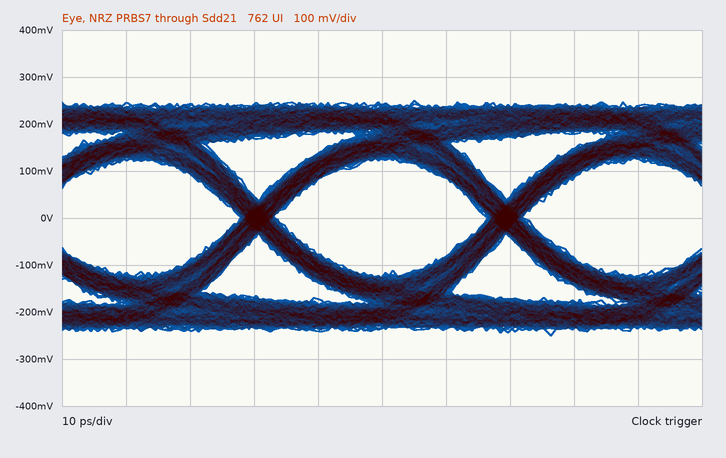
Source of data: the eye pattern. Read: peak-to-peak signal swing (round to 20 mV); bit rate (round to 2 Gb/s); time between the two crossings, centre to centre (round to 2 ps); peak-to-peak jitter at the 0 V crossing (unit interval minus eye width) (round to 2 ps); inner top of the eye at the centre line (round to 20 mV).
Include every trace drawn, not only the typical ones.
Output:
500 mV
26 Gb/s
38 ps
6 ps
120 mV
